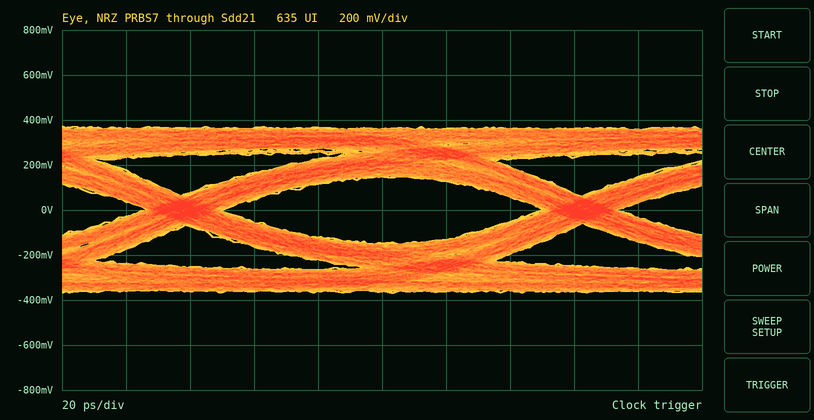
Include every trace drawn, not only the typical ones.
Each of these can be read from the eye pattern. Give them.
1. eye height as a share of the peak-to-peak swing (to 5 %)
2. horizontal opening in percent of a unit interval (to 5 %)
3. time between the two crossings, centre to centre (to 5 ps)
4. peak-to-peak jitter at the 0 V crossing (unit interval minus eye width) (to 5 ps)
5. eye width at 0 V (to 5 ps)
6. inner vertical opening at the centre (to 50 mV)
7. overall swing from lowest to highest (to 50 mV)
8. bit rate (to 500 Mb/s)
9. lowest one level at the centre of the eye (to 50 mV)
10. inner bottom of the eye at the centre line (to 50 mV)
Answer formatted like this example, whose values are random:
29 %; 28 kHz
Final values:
40 %; 80 %; 125 ps; 25 ps; 100 ps; 300 mV; 750 mV; 8.0 Gb/s; 150 mV; -150 mV
